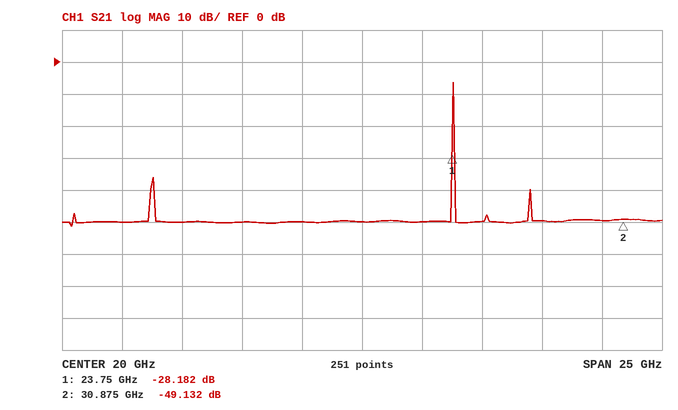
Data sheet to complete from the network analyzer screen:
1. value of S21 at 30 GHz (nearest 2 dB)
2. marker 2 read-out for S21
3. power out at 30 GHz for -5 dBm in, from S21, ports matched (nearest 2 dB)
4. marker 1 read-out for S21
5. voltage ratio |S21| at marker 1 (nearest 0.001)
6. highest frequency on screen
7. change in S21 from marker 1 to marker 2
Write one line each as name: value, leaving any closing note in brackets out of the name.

value of S21 at 30 GHz: -50 dB
marker 2 read-out for S21: -49.132 dB
power out at 30 GHz for -5 dBm in, from S21, ports matched: -54 dBm
marker 1 read-out for S21: -28.182 dB
voltage ratio |S21| at marker 1: 0.039
highest frequency on screen: 32.5 GHz
change in S21 from marker 1 to marker 2: -20.950 dB
